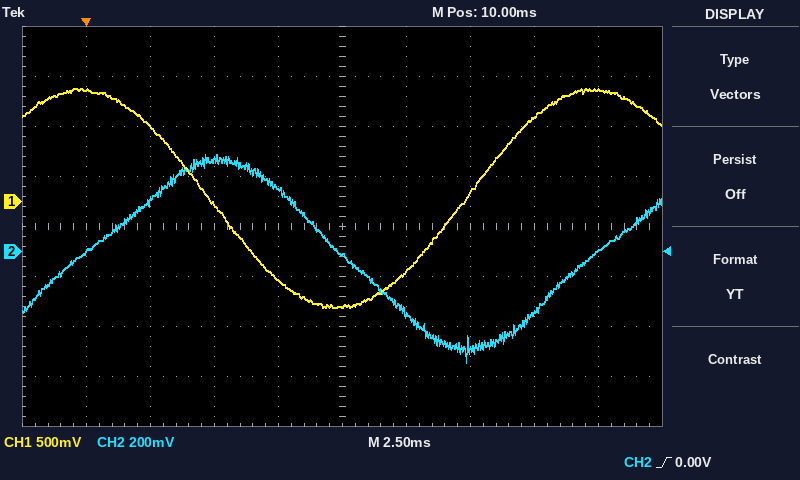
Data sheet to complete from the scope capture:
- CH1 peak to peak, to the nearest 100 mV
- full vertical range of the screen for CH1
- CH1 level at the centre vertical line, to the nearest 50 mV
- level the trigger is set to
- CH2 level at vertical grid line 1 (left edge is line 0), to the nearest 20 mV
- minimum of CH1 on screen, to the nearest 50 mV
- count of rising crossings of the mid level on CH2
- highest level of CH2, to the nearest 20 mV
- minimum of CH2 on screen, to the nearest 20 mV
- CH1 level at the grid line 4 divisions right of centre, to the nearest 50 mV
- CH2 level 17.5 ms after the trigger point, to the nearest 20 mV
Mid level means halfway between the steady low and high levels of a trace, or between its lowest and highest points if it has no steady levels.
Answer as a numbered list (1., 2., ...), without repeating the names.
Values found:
1. 2.20 V
2. 4 V
3. -1.05 V
4. 0.00 V
5. 0 mV
6. -1.05 V
7. 2
8. 380 mV
9. -440 mV
10. 1.10 V
11. -240 mV
